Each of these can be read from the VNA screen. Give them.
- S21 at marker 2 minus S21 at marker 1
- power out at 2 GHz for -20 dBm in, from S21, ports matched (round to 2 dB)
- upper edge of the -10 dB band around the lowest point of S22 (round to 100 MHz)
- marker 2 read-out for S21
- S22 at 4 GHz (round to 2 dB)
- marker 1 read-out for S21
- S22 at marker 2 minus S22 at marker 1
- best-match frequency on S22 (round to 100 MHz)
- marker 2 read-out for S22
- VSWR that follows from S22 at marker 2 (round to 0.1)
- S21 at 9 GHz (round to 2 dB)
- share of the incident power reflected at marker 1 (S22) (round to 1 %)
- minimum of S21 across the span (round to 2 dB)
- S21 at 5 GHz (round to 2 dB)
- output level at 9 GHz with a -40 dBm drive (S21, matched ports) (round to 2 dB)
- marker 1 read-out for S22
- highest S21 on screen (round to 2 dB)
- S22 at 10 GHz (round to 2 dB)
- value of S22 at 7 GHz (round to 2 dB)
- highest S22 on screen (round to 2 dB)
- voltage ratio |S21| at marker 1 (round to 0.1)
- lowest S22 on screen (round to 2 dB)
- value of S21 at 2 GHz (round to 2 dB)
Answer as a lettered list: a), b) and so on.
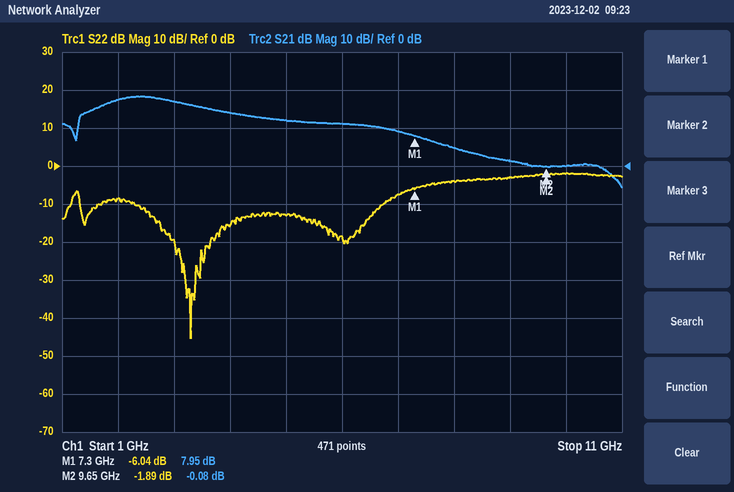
a) -8.03 dB
b) -2 dBm
c) 6.7 GHz
d) -0.08 dB
e) -16 dB
f) 7.95 dB
g) 4.15 dB
h) 3.3 GHz
i) -1.89 dB
j) 9.2
k) 2 dB
l) 25 %
m) -6 dB
n) 12 dB
o) -38 dBm
p) -6.04 dB
q) 18 dB
r) -2 dB
s) -8 dB
t) -2 dB
u) 2.5
v) -46 dB
w) 18 dB
